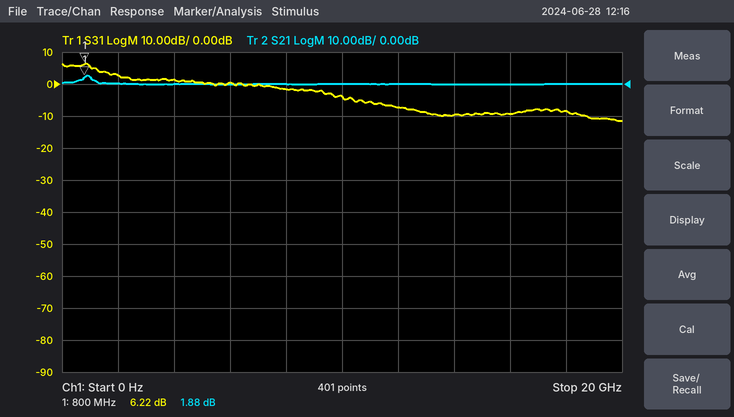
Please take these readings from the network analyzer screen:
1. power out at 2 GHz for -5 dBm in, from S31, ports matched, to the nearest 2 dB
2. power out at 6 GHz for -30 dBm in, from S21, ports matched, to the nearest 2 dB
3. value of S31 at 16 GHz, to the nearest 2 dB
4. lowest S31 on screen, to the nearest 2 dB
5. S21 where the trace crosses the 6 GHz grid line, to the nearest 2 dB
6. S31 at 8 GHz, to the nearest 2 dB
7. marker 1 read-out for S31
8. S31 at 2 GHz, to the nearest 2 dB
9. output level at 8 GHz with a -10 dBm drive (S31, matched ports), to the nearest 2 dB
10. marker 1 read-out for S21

-2 dBm
-30 dBm
-10 dB
-12 dB
0 dB
-2 dB
6.22 dB
2 dB
-12 dBm
1.88 dB
